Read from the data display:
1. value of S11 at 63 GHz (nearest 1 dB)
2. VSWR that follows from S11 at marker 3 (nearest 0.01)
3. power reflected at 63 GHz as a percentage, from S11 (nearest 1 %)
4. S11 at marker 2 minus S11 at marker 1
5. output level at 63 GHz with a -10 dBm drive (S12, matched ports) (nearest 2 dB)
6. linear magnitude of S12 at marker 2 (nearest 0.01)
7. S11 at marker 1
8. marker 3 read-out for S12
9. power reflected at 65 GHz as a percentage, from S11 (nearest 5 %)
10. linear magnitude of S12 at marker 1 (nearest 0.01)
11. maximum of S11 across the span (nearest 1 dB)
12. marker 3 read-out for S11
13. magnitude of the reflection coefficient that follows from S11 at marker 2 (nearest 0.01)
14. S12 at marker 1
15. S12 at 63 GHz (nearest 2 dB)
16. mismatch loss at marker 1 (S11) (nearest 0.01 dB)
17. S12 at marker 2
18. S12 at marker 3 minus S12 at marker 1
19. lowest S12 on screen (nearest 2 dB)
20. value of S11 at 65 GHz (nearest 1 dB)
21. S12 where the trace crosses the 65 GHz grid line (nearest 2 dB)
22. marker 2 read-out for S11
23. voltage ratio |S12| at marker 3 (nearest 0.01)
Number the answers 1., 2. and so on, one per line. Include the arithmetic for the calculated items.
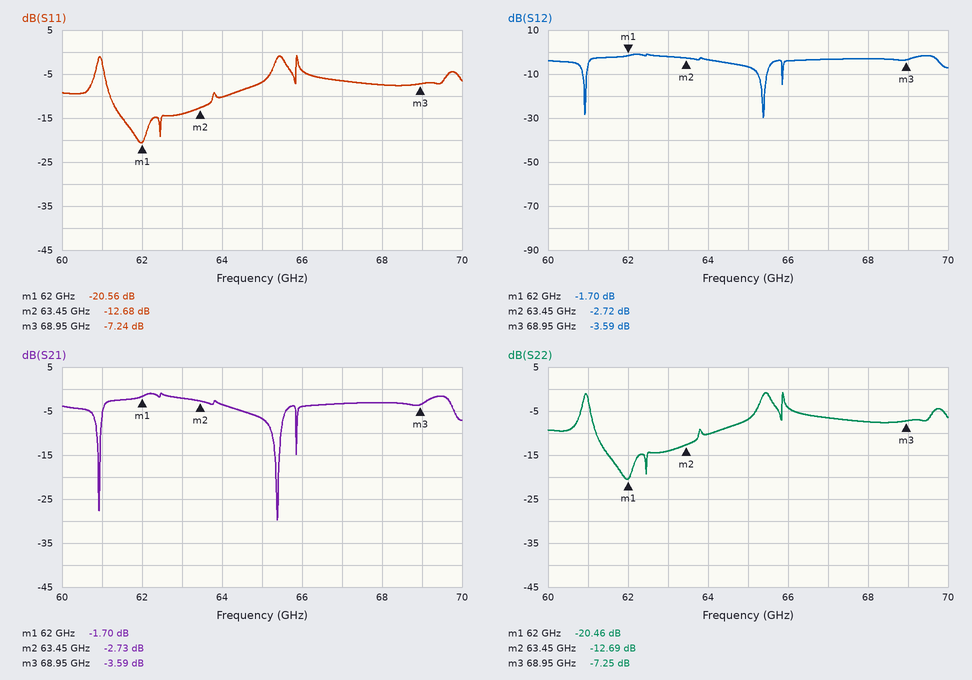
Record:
1. -14 dB
2. (1 + 0.4345)/(1 − 0.4345) ≈ 2.54
3. 10^(-14/10) ≈ 4 %
4. -12.68 − (-20.56) = 7.88 dB
5. -10 dBm + (-2 dB) = -12 dBm
6. 10^(-2.72/20) ≈ 0.73
7. -20.56 dB
8. -3.59 dB
9. 10^(-7/10) ≈ 20 %
10. 10^(-1.7/20) ≈ 0.82
11. -1 dB
12. -7.24 dB
13. 10^(-12.68/20) ≈ 0.23
14. -1.70 dB
15. -2 dB
16. −10 log10(1 − 10^(-20.56/10)) ≈ 0.04 dB
17. -2.72 dB
18. -3.59 − (-1.7) = -1.89 dB
19. -30 dB
20. -7 dB
21. -6 dB
22. -12.68 dB
23. 10^(-3.59/20) ≈ 0.66
